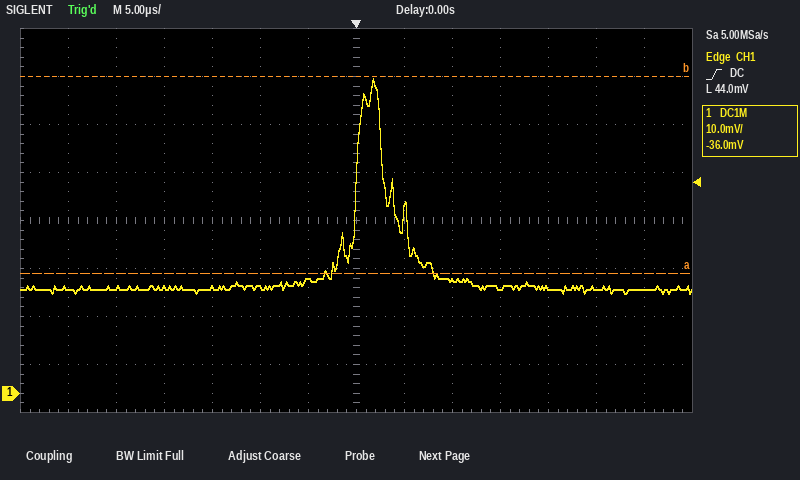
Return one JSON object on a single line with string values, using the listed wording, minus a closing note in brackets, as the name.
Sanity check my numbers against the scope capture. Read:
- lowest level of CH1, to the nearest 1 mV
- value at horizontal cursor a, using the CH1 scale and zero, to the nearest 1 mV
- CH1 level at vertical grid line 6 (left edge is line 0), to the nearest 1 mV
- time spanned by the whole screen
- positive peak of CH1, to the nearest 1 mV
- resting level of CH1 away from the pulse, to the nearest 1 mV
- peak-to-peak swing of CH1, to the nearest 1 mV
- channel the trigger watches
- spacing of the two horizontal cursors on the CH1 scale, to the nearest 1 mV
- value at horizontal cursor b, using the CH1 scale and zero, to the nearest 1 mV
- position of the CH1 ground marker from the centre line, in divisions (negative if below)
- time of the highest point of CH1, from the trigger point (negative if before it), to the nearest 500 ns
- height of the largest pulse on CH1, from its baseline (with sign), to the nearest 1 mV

{"lowest level of CH1, to the nearest 1 mV": "21 mV", "value at horizontal cursor a, using the CH1 scale and zero, to the nearest 1 mV": "25 mV", "CH1 level at vertical grid line 6 (left edge is line 0), to the nearest 1 mV": "24 mV", "time spanned by the whole screen": "70 µs", "positive peak of CH1, to the nearest 1 mV": "66 mV", "resting level of CH1 away from the pulse, to the nearest 1 mV": "22 mV", "peak-to-peak swing of CH1, to the nearest 1 mV": "45 mV", "channel the trigger watches": "CH1", "spacing of the two horizontal cursors on the CH1 scale, to the nearest 1 mV": "41 mV", "value at horizontal cursor b, using the CH1 scale and zero, to the nearest 1 mV": "66 mV", "position of the CH1 ground marker from the centre line, in divisions": "-3.6 div", "time of the highest point of CH1, from the trigger point (negative if before it), to the nearest 500 ns": "+2.0 µs", "height of the largest pulse on CH1, from its baseline (with sign), to the nearest 1 mV": "+44 mV"}
